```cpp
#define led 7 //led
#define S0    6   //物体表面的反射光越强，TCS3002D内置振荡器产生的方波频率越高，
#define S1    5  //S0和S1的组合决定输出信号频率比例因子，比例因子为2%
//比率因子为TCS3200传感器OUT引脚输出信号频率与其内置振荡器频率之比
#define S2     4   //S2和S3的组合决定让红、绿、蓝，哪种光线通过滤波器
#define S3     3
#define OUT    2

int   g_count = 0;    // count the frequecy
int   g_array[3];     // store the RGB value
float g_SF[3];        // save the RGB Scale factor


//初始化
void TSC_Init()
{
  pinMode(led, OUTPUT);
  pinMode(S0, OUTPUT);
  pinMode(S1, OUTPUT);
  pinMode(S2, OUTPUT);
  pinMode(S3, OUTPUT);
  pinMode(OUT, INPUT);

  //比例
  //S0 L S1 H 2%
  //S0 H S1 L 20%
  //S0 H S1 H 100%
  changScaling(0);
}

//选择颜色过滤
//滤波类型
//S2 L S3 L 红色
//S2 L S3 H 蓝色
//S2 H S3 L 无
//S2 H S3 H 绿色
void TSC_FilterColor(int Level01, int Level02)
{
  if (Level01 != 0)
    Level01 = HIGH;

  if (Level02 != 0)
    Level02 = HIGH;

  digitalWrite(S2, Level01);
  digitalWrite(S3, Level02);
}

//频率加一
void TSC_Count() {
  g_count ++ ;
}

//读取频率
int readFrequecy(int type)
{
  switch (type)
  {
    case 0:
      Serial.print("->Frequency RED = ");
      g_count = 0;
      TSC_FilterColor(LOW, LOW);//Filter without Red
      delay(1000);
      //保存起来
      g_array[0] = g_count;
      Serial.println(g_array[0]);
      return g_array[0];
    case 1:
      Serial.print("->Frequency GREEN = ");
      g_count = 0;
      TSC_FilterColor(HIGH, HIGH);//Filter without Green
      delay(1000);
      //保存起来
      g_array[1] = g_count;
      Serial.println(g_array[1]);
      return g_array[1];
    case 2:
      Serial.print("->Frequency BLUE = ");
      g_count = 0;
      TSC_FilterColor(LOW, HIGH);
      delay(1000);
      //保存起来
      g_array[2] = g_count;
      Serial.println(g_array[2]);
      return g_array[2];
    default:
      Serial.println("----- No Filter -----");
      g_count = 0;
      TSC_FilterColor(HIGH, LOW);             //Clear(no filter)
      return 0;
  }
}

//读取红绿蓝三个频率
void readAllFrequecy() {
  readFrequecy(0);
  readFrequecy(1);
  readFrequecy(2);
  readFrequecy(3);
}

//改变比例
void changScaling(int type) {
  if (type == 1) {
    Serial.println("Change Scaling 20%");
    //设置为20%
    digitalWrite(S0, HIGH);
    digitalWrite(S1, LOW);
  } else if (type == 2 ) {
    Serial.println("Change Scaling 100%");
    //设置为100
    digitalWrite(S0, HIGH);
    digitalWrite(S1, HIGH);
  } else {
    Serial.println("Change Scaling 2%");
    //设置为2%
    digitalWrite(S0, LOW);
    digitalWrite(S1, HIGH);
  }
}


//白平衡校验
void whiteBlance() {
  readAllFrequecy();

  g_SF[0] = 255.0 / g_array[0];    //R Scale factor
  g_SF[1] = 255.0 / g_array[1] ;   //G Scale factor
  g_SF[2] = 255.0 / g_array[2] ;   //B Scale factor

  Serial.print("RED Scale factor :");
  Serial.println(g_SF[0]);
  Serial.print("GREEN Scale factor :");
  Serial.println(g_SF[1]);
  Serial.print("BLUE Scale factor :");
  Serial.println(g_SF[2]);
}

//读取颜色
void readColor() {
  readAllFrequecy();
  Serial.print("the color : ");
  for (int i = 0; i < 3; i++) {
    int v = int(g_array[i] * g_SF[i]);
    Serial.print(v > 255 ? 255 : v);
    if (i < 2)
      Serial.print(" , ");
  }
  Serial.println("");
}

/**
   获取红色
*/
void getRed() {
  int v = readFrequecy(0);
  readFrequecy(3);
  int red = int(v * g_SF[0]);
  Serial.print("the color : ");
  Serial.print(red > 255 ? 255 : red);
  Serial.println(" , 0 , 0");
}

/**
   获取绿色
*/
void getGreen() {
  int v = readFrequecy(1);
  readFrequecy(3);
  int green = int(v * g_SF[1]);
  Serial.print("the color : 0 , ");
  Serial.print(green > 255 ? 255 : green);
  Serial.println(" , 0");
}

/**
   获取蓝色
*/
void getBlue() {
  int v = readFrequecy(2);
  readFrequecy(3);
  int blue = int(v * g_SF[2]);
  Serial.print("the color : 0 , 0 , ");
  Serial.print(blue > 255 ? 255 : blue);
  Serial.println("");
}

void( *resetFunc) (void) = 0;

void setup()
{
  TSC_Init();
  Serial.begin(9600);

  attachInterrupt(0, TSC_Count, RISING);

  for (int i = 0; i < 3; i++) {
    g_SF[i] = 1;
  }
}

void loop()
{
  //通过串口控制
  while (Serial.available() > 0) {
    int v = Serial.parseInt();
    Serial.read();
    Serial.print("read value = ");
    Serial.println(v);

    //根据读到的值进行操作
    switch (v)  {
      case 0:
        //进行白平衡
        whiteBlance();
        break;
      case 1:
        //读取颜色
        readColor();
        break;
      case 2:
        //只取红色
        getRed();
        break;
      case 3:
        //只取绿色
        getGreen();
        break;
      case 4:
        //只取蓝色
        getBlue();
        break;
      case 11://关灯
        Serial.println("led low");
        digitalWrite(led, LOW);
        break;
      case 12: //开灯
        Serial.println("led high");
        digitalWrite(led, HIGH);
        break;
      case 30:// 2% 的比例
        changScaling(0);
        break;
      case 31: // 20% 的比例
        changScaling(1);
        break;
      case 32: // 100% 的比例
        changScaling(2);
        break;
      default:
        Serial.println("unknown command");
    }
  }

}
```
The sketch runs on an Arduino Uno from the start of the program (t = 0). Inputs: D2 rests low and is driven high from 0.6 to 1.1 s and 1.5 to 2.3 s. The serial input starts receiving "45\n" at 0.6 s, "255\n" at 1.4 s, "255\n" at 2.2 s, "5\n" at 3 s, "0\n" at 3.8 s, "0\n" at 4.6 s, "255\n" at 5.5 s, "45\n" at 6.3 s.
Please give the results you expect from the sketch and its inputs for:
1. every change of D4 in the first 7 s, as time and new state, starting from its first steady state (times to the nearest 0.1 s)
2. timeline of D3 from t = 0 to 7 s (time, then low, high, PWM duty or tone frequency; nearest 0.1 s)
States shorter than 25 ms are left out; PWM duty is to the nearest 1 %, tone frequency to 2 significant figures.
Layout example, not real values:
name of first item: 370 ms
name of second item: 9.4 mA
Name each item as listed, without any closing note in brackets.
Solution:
every change of D4 in the first 7 s, as time and new state, starting from its first steady state: 0 s low; 4.8 s high; 5.8 s low; 6.8 s high; 6.9 s low
timeline of D3 from t = 0 to 7 s: 0 s low; 4.8 s high; 6.8 s low
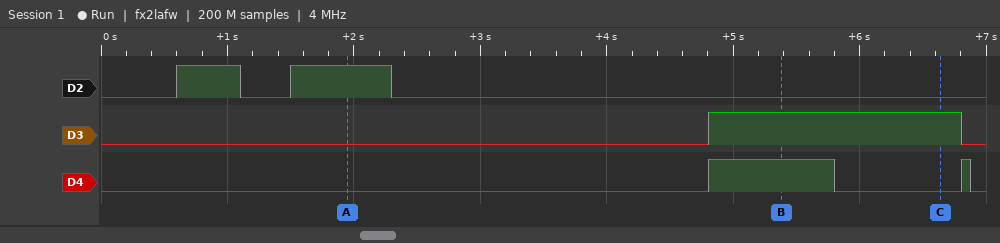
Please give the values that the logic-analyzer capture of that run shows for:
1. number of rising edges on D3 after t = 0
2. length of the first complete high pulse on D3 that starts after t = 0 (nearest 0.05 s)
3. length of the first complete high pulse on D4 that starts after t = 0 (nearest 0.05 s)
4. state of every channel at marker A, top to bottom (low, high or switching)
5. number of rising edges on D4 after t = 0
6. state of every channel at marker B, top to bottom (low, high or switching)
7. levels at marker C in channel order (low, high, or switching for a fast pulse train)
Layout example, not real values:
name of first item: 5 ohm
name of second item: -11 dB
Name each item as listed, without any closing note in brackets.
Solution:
number of rising edges on D3 after t = 0: 1
length of the first complete high pulse on D3 that starts after t = 0: 2.00 s
length of the first complete high pulse on D4 that starts after t = 0: 1.00 s
state of every channel at marker A, top to bottom: D2 high, D3 low, D4 low
number of rising edges on D4 after t = 0: 2
state of every channel at marker B, top to bottom: D2 low, D3 high, D4 high
levels at marker C in channel order: D2 low, D3 high, D4 low
